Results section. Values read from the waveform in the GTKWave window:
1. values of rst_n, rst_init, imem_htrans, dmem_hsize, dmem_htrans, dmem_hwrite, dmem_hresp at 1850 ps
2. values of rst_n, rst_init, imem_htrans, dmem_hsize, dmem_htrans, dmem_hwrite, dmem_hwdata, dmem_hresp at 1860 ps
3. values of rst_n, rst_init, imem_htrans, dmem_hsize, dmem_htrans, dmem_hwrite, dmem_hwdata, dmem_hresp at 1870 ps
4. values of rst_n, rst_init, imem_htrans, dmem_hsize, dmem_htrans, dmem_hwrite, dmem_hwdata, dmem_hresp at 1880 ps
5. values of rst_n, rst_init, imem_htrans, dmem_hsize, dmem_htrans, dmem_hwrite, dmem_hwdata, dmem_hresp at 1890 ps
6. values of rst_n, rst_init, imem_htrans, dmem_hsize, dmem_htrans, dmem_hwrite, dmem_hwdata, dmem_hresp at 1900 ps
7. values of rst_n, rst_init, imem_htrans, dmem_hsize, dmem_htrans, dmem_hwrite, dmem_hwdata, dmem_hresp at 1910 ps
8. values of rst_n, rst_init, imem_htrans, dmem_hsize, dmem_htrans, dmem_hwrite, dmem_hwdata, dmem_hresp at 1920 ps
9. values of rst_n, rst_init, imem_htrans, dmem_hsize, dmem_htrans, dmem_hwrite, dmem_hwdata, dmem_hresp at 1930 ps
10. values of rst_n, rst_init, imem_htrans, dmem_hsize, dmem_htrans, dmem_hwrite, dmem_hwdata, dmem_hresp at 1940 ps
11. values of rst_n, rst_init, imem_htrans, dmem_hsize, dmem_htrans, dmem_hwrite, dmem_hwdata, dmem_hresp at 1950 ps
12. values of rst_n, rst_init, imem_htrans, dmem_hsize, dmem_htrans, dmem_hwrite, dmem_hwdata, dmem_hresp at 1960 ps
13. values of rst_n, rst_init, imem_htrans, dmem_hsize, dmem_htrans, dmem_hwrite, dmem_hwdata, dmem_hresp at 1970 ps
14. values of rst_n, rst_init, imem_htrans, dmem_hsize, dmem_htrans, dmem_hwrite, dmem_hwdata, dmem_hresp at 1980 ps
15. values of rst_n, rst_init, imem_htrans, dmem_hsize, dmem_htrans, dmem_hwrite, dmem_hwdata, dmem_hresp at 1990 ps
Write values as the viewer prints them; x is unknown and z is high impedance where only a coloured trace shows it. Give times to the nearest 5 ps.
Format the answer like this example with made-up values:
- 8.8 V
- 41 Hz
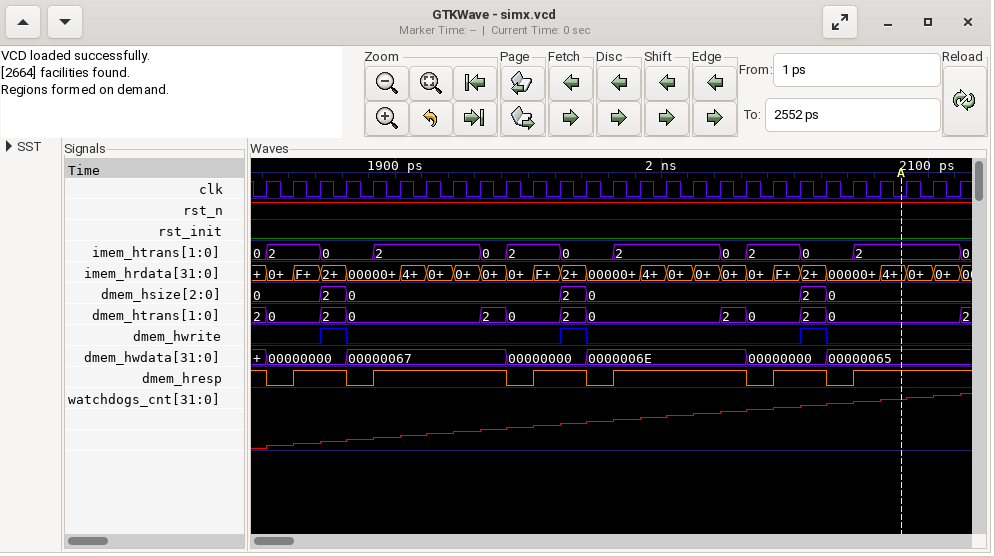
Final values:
- rst_n=1, rst_init=0, imem_htrans=0, dmem_hsize=0, dmem_htrans=2, dmem_hwrite=0, dmem_hresp=1
- rst_n=1, rst_init=0, imem_htrans=2, dmem_hsize=0, dmem_htrans=0, dmem_hwrite=0, dmem_hwdata=00000000, dmem_hresp=0
- rst_n=1, rst_init=0, imem_htrans=2, dmem_hsize=0, dmem_htrans=0, dmem_hwrite=0, dmem_hwdata=00000000, dmem_hresp=1
- rst_n=1, rst_init=0, imem_htrans=0, dmem_hsize=2, dmem_htrans=2, dmem_hwrite=1, dmem_hwdata=00000000, dmem_hresp=1
- rst_n=1, rst_init=0, imem_htrans=0, dmem_hsize=0, dmem_htrans=0, dmem_hwrite=0, dmem_hwdata=00000067, dmem_hresp=0
- rst_n=1, rst_init=0, imem_htrans=2, dmem_hsize=0, dmem_htrans=0, dmem_hwrite=0, dmem_hwdata=00000067, dmem_hresp=1
- rst_n=1, rst_init=0, imem_htrans=2, dmem_hsize=0, dmem_htrans=0, dmem_hwrite=0, dmem_hwdata=00000067, dmem_hresp=1
- rst_n=1, rst_init=0, imem_htrans=2, dmem_hsize=0, dmem_htrans=0, dmem_hwrite=0, dmem_hwdata=00000067, dmem_hresp=1
- rst_n=1, rst_init=0, imem_htrans=2, dmem_hsize=0, dmem_htrans=0, dmem_hwrite=0, dmem_hwdata=00000067, dmem_hresp=1
- rst_n=1, rst_init=0, imem_htrans=0, dmem_hsize=0, dmem_htrans=2, dmem_hwrite=0, dmem_hwdata=00000067, dmem_hresp=1
- rst_n=1, rst_init=0, imem_htrans=2, dmem_hsize=0, dmem_htrans=0, dmem_hwrite=0, dmem_hwdata=00000000, dmem_hresp=0
- rst_n=1, rst_init=0, imem_htrans=2, dmem_hsize=0, dmem_htrans=0, dmem_hwrite=0, dmem_hwdata=00000000, dmem_hresp=1
- rst_n=1, rst_init=0, imem_htrans=0, dmem_hsize=2, dmem_htrans=2, dmem_hwrite=1, dmem_hwdata=00000000, dmem_hresp=1
- rst_n=1, rst_init=0, imem_htrans=0, dmem_hsize=0, dmem_htrans=0, dmem_hwrite=0, dmem_hwdata=0000006E, dmem_hresp=0
- rst_n=1, rst_init=0, imem_htrans=2, dmem_hsize=0, dmem_htrans=0, dmem_hwrite=0, dmem_hwdata=0000006E, dmem_hresp=1
